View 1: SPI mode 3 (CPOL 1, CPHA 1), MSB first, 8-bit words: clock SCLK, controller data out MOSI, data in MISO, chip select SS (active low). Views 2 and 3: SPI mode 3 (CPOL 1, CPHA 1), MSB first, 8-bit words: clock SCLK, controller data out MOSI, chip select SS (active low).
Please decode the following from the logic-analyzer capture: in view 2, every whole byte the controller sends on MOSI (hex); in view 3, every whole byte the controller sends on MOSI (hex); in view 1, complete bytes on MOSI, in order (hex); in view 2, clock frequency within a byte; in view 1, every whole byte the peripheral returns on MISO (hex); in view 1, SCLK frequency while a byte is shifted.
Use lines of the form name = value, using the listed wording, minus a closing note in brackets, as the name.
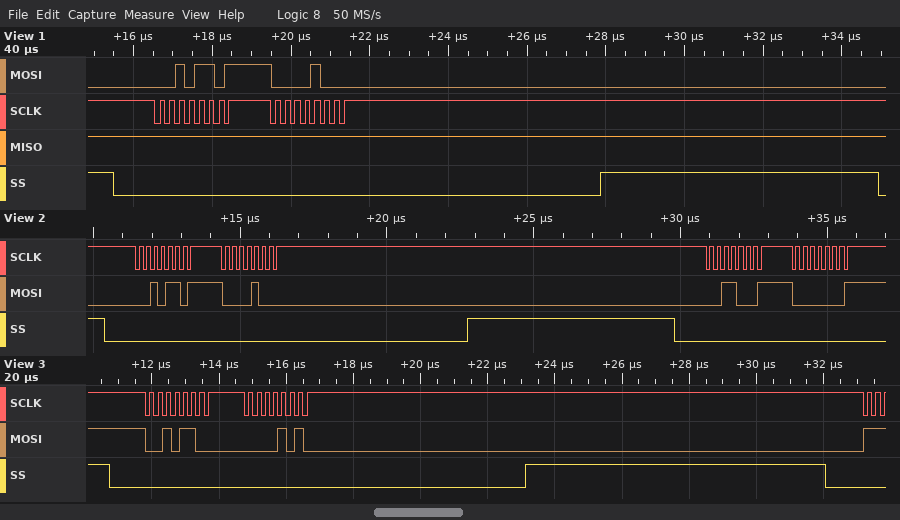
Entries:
in view 2, every whole byte the controller sends on MOSI = 2D 08 31 01
in view 3, every whole byte the controller sends on MOSI = 2C 0A
in view 1, complete bytes on MOSI, in order = 2D 08
in view 2, clock frequency within a byte = 4 MHz
in view 1, every whole byte the peripheral returns on MISO = FF FF
in view 1, SCLK frequency while a byte is shifted = 4 MHz
